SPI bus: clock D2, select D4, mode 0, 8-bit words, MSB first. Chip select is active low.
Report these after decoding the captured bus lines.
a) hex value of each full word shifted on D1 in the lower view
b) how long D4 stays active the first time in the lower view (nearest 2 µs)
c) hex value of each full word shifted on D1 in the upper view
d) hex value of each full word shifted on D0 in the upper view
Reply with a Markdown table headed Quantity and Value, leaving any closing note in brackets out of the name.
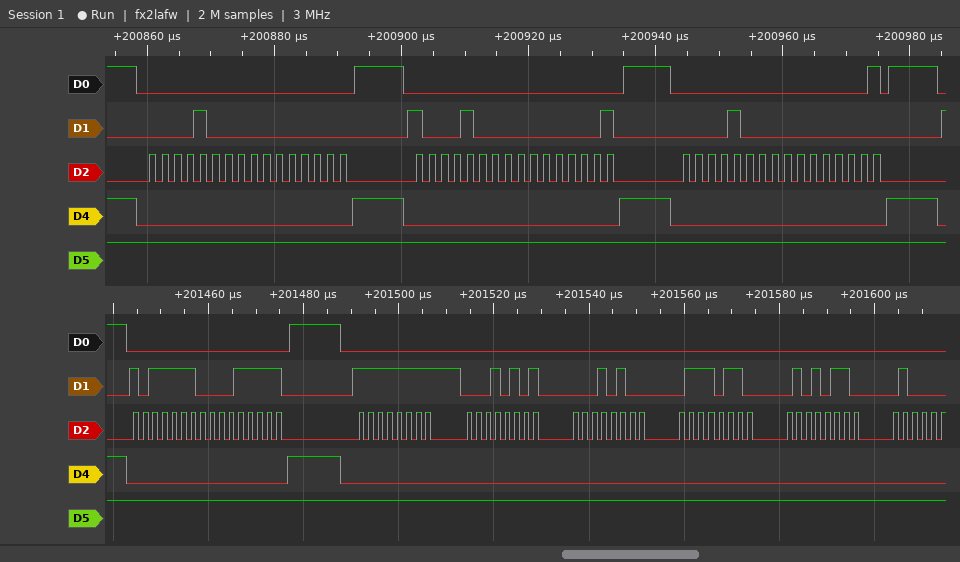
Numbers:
| Quantity | Value |
|---|---|
| hex value of each full word shifted on D1 in the lower view | BE, 1F, FF, 15, 14, 76, 56 |
| how long D4 stays active the first time in the lower view | 34 µs |
| hex value of each full word shifted on D1 in the upper view | 08, 00, 88, 01, 08, 00 |
| hex value of each full word shifted on D0 in the upper view | 00, 00, 00, 00, 00, 01 |
